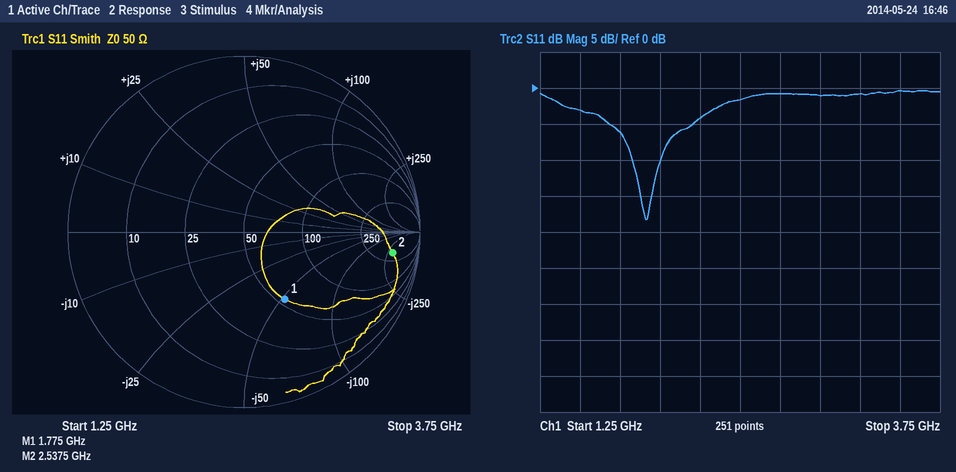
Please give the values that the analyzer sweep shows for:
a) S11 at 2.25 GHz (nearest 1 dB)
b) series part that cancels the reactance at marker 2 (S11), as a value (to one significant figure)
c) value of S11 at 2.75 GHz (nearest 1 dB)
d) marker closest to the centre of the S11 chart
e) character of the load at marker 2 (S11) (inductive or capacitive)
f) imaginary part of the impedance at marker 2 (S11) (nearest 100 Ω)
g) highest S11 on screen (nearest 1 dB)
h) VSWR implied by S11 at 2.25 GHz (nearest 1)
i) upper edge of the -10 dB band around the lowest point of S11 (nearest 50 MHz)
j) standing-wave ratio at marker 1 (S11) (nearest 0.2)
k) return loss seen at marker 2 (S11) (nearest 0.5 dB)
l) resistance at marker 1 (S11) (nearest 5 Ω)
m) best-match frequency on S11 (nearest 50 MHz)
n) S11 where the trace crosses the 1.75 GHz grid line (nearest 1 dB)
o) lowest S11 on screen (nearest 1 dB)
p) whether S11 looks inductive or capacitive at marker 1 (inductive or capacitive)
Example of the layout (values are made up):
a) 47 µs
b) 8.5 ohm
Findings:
a) -4 dB
b) 20 nH
c) -1 dB
d) marker 1
e) capacitive
f) -300 Ω
g) 0 dB
h) 4
i) 2.00 GHz
j) 2.6
k) 1.5 dB
l) 55 Ω
m) 1.90 GHz
n) -6 dB
o) -18 dB
p) capacitive
